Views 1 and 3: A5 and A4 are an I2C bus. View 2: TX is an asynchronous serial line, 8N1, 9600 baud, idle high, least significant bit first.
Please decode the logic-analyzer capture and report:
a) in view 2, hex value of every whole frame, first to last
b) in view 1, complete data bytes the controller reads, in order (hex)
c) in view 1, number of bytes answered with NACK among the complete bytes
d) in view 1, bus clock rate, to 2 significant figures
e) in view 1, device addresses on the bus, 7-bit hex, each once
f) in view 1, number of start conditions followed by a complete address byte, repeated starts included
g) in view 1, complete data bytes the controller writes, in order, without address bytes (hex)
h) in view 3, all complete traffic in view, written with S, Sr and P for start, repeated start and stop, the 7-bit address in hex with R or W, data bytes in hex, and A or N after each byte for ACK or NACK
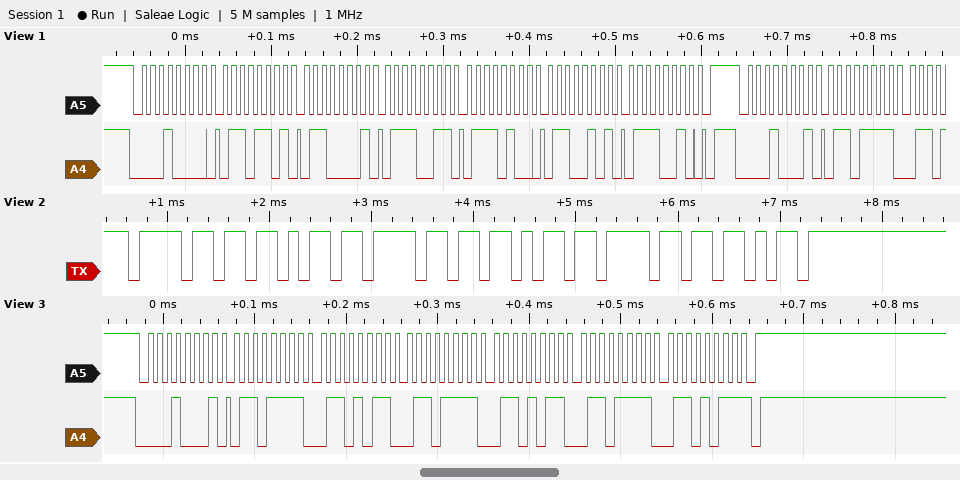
0x6F 0x6B 0x6F 0x6B 0x6F 0x6B
6F
0
100 kHz
0x08
2
6D 61 73 74 65 72
S 08R A 6F A 6B A 6F A 6B A 6F A 6B N P
